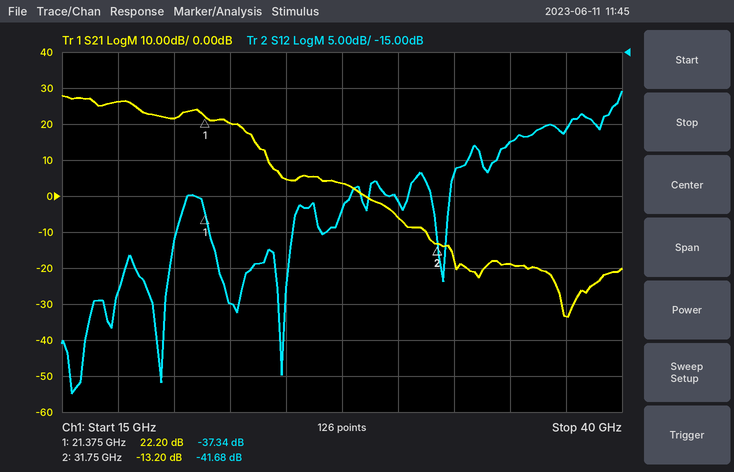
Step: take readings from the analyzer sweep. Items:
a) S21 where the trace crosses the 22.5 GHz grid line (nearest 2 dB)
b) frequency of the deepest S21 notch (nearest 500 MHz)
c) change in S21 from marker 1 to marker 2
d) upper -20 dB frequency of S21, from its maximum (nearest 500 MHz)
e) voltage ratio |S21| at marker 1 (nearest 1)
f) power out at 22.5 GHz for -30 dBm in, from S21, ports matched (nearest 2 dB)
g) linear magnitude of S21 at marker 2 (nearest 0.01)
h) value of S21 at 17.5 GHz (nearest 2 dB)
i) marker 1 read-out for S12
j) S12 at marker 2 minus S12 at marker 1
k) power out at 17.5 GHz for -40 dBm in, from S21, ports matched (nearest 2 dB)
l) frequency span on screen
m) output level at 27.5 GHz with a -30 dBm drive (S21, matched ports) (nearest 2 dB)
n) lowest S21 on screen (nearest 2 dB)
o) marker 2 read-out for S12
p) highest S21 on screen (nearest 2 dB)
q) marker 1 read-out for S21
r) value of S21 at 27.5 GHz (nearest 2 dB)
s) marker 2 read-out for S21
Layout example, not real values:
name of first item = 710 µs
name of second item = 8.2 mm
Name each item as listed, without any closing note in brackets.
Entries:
S21 where the trace crosses the 22.5 GHz grid line = 20 dB
frequency of the deepest S21 notch = 37.5 GHz
change in S21 from marker 1 to marker 2 = -35.40 dB
upper -20 dB frequency of S21, from its maximum = 24.5 GHz
voltage ratio |S21| at marker 1 = 13
power out at 22.5 GHz for -30 dBm in, from S21, ports matched = -10 dBm
linear magnitude of S21 at marker 2 = 0.22
value of S21 at 17.5 GHz = 26 dB
marker 1 read-out for S12 = -37.34 dB
S12 at marker 2 minus S12 at marker 1 = -4.34 dB
power out at 17.5 GHz for -40 dBm in, from S21, ports matched = -14 dBm
frequency span on screen = 25 GHz
output level at 27.5 GHz with a -30 dBm drive (S21, matched ports) = -26 dBm
lowest S21 on screen = -34 dB
marker 2 read-out for S12 = -41.68 dB
highest S21 on screen = 28 dB
marker 1 read-out for S21 = 22.20 dB
value of S21 at 27.5 GHz = 4 dB
marker 2 read-out for S21 = -13.20 dB
